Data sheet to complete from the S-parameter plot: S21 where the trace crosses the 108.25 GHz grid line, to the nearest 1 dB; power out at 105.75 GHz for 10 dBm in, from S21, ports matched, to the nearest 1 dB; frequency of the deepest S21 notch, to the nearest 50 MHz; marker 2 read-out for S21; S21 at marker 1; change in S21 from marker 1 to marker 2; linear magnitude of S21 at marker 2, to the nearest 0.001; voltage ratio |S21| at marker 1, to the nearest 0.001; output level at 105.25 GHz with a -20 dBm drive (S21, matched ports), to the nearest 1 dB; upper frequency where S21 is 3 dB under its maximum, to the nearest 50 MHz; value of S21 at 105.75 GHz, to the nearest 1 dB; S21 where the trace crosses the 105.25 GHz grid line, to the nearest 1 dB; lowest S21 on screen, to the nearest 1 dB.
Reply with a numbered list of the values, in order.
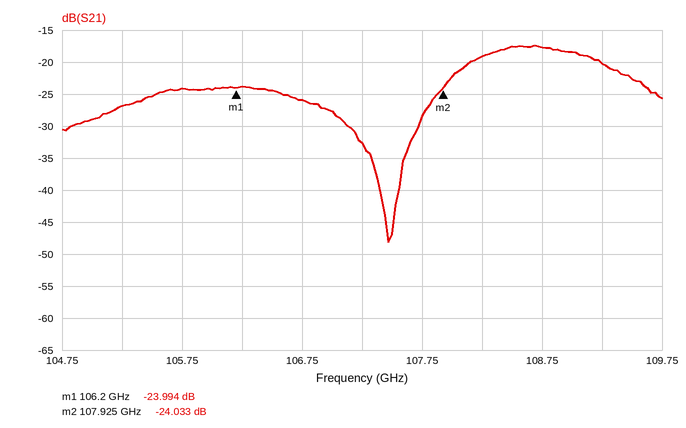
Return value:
1. -19 dB
2. -14 dBm
3. 107.45 GHz
4. -24.033 dB
5. -23.994 dB
6. -0.039 dB
7. 0.063
8. 0.063
9. -47 dBm
10. 109.25 GHz
11. -24 dB
12. -27 dB
13. -48 dB
